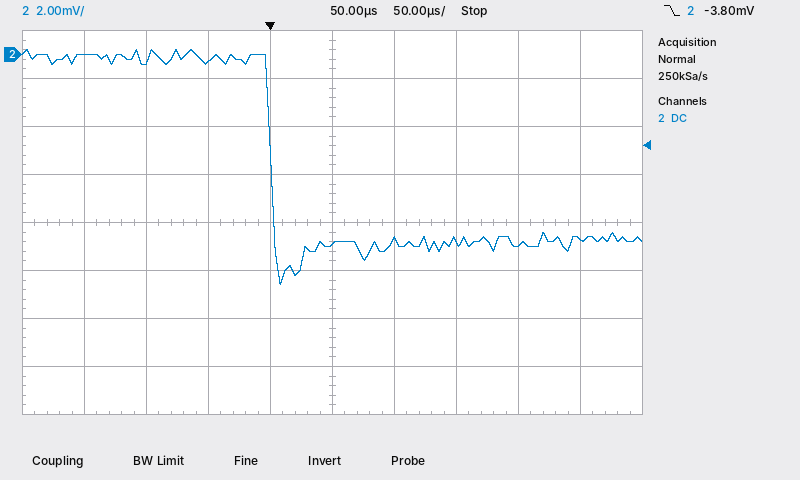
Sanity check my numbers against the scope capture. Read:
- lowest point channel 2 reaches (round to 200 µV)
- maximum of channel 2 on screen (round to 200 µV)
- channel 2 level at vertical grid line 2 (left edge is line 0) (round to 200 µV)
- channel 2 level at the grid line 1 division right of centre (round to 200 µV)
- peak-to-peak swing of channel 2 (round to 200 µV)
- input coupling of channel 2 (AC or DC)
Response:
-9.6 mV
200 µV
-200 µV
-7.8 mV
9.8 mV
DC
